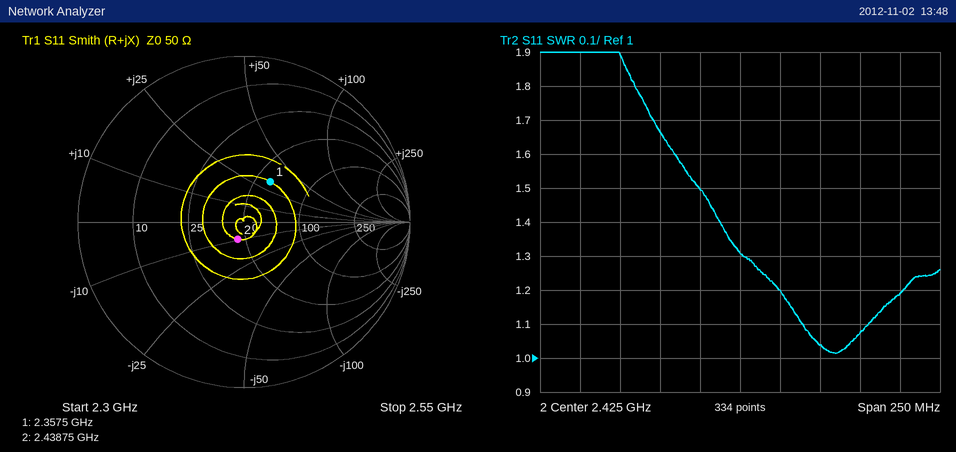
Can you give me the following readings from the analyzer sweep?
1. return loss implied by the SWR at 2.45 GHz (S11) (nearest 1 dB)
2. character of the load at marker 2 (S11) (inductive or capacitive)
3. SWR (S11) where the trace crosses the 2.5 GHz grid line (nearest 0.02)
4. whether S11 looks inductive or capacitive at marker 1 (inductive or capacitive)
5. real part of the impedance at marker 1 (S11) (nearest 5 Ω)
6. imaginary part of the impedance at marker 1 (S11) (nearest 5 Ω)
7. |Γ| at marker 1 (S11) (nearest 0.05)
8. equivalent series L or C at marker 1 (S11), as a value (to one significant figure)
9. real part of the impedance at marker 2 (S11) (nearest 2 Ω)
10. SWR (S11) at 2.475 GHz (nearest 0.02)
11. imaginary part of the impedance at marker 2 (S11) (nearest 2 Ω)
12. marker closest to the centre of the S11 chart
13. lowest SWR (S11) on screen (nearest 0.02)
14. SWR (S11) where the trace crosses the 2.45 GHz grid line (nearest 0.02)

21 dB
capacitive
1.08
inductive
60 Ω
+30 Ω
0.30
2 nH
46 Ω
1.04
-10 Ω
marker 2
1.02
1.20
